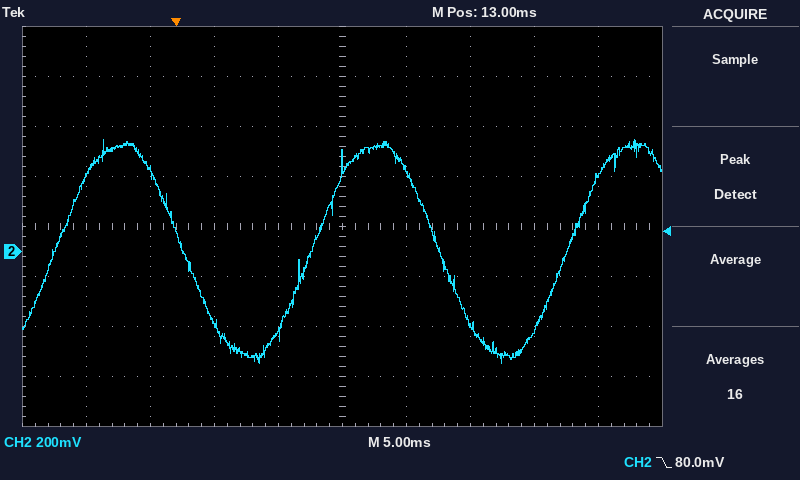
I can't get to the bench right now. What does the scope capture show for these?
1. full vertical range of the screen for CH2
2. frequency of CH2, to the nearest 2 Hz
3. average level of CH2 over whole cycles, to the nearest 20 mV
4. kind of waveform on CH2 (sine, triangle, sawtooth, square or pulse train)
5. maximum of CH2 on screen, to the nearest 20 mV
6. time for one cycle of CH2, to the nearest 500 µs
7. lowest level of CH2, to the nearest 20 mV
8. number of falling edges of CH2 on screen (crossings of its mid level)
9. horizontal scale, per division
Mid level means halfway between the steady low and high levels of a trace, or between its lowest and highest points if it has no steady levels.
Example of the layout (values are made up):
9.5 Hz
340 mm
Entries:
1.6 V
50 Hz
0 mV
sine
440 mV
20.0 ms
-440 mV
2
5 ms
